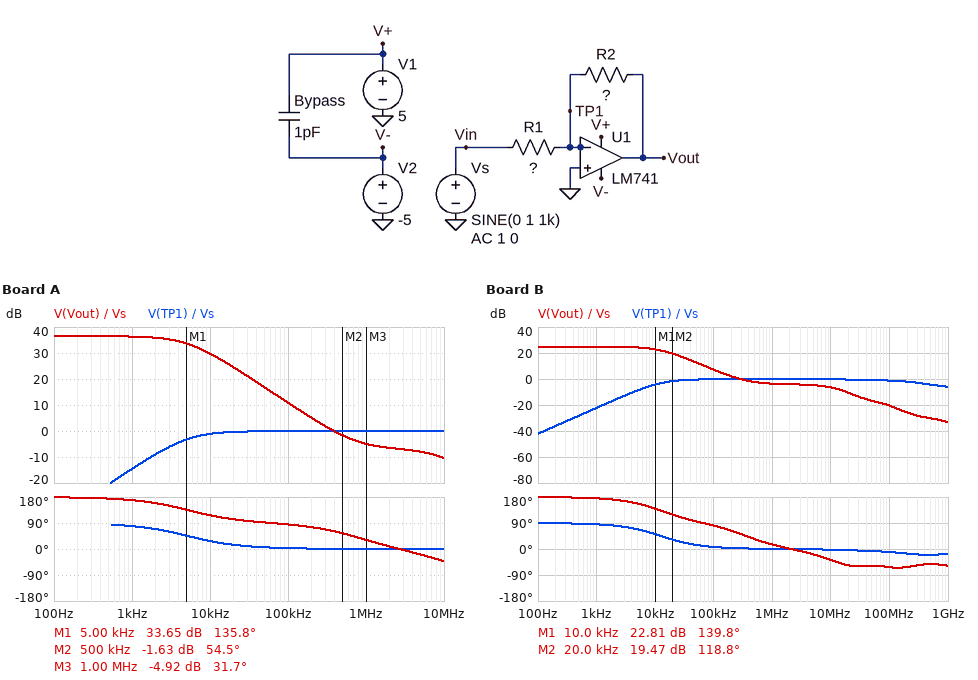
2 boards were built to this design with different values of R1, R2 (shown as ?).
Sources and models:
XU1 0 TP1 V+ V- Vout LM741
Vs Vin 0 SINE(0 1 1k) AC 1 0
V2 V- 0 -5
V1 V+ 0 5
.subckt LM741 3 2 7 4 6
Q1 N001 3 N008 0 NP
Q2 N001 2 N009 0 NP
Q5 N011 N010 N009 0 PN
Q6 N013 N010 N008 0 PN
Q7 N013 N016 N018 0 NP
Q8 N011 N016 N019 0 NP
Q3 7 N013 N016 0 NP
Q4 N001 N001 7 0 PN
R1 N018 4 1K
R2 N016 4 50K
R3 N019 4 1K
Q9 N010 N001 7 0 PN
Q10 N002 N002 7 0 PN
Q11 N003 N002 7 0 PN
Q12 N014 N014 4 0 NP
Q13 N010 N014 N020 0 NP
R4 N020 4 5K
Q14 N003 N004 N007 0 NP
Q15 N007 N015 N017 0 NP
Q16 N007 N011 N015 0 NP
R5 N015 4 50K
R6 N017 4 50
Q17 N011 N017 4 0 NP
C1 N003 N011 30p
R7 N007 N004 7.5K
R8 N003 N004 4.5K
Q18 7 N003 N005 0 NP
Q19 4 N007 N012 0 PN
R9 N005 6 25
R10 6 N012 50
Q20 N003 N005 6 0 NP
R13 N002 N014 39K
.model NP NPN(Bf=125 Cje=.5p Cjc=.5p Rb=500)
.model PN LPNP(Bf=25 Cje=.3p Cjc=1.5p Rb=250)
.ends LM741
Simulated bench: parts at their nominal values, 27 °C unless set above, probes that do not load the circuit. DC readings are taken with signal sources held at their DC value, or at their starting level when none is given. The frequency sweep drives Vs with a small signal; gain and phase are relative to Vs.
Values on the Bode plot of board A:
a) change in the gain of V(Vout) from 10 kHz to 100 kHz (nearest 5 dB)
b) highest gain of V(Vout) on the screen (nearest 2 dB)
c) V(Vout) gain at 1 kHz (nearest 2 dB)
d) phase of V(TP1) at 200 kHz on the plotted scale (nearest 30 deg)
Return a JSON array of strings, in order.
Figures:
["-20 dB", "36 dB", "36 dB", "0 deg"]
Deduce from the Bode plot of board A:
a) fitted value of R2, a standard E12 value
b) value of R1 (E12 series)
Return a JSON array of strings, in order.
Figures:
["22 kΩ", "330 Ω"]
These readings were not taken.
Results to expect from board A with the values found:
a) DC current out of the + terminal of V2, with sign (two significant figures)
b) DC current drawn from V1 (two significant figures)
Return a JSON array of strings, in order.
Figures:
["-460 µA", "460 µA"]
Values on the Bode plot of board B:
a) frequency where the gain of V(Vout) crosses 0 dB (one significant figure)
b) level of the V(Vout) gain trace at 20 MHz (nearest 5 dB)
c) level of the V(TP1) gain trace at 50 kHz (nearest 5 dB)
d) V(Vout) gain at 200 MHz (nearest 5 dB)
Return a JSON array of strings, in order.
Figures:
["300 kHz", "-10 dB", "0 dB", "-25 dB"]
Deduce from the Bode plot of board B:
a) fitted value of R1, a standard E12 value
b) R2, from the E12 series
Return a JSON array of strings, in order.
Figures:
["680 Ω", "12 kΩ"]
